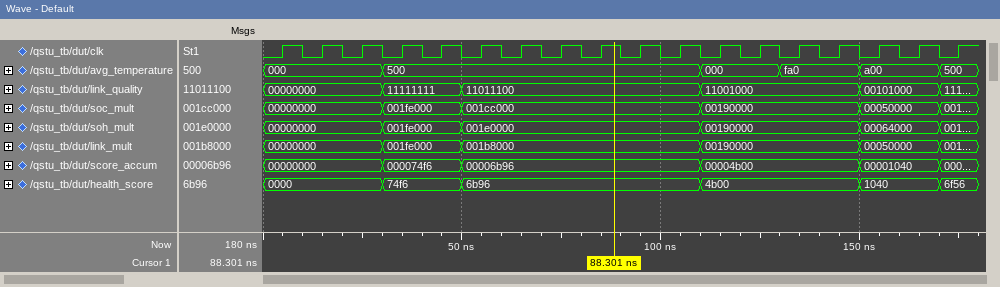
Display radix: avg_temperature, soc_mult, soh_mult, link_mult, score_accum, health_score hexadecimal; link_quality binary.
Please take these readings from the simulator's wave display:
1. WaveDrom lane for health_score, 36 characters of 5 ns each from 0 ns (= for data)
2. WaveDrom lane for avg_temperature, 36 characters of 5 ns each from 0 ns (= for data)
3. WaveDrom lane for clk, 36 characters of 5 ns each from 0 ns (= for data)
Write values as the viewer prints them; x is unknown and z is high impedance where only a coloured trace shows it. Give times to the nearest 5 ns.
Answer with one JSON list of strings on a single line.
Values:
["{name: 'health_score', wave: '=.....=...=...........=.......=...=.', data: '0000 74f6 6b96 4b00 1040 6f56'}", "{name: 'avg_temperature', wave: '=.....=...............=...=...=...=.', data: '000 500 000 fa0 a00 500'}", "{name: 'clk', wave: '010101010101010101010101010101010101'}"]
